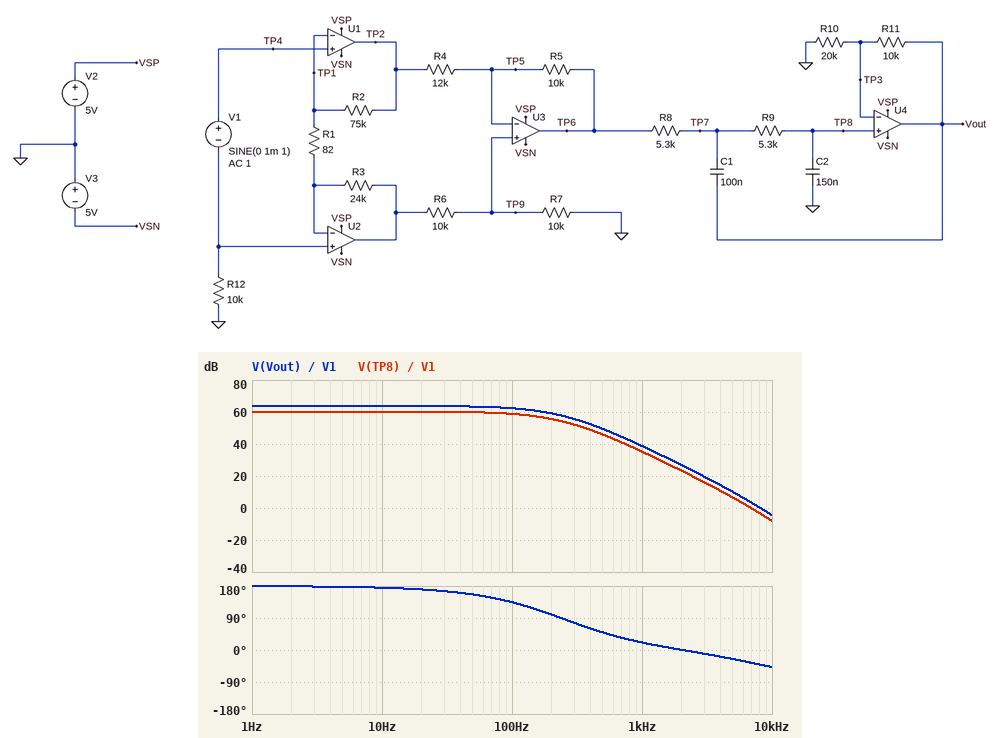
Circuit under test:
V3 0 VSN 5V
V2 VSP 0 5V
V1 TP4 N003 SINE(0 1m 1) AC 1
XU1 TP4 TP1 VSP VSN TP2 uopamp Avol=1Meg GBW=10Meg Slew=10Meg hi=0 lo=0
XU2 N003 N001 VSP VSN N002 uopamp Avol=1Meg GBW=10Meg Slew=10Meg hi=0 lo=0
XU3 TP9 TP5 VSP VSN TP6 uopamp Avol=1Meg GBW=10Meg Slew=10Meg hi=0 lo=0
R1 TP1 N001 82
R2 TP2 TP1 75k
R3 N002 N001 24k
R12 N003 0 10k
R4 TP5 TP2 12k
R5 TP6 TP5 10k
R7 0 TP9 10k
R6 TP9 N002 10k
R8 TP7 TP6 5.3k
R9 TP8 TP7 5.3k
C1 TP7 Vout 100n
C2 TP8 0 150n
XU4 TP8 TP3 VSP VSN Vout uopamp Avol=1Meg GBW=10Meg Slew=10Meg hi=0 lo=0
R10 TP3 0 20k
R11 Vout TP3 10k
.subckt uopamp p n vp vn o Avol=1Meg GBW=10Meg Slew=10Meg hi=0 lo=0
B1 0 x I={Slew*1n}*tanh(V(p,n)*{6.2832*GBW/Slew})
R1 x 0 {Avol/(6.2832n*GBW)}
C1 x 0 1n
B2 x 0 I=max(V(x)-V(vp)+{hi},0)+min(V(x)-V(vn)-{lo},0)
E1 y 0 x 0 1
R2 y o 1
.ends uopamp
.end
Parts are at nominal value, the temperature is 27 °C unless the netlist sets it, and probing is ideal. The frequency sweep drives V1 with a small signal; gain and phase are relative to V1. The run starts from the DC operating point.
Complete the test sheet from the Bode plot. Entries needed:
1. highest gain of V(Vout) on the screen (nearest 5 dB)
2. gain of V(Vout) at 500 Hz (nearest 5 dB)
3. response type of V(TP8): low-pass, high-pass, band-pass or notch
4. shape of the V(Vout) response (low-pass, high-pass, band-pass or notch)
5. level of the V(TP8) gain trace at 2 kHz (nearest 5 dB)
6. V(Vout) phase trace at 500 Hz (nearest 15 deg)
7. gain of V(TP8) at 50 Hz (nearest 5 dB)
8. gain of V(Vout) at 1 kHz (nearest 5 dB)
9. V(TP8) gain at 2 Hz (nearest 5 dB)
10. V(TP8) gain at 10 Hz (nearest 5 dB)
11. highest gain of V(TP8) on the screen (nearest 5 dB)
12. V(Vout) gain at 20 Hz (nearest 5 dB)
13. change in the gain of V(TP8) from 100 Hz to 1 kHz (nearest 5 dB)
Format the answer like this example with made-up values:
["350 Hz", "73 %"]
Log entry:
["65 dB", "50 dB", "low-pass", "low-pass", "25 dB", "45 deg", "60 dB", "40 dB", "60 dB", "60 dB", "60 dB", "65 dB", "-25 dB"]
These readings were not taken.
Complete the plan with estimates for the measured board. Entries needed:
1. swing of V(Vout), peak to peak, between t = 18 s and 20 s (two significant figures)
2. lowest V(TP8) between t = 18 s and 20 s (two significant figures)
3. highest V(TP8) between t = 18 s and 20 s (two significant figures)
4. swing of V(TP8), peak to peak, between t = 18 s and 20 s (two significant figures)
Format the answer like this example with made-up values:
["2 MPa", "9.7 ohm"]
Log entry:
["3.1 V", "-1.0 V", "1.0 V", "2.1 V"]
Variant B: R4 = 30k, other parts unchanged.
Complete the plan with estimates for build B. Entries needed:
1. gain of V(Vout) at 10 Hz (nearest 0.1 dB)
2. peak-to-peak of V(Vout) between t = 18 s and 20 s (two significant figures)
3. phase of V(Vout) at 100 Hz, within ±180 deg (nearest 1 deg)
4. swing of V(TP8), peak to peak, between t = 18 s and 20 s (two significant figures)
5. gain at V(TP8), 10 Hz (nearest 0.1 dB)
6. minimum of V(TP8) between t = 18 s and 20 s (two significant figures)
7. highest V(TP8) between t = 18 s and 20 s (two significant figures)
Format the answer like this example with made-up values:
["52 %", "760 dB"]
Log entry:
["57.5 dB", "1.5 V", "134 deg", "1.0 V", "54.0 dB", "-500 mV", "500 mV"]
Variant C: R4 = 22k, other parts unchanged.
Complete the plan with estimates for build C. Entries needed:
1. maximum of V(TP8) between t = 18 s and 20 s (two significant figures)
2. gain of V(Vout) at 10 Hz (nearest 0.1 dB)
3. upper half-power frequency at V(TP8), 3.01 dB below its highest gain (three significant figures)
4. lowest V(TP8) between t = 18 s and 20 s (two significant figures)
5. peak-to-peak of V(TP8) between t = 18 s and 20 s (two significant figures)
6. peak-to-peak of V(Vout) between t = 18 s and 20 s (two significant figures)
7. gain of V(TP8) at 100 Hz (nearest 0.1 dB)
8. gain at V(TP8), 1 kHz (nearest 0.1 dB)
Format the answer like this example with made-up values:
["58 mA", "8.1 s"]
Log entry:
["630 mV", "59.5 dB", "153 Hz", "-630 mV", "1.3 V", "1.9 V", "54.5 dB", "30.9 dB"]
